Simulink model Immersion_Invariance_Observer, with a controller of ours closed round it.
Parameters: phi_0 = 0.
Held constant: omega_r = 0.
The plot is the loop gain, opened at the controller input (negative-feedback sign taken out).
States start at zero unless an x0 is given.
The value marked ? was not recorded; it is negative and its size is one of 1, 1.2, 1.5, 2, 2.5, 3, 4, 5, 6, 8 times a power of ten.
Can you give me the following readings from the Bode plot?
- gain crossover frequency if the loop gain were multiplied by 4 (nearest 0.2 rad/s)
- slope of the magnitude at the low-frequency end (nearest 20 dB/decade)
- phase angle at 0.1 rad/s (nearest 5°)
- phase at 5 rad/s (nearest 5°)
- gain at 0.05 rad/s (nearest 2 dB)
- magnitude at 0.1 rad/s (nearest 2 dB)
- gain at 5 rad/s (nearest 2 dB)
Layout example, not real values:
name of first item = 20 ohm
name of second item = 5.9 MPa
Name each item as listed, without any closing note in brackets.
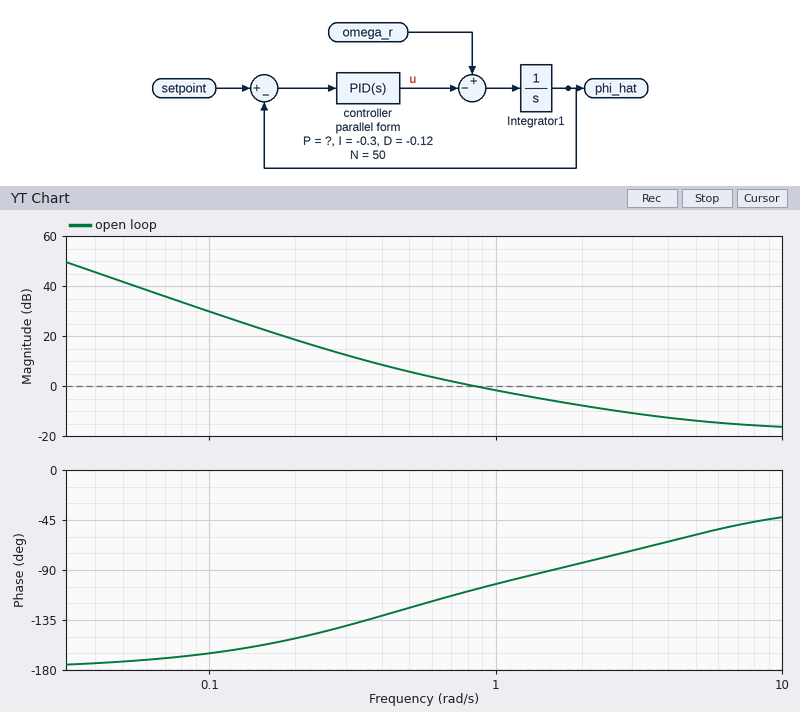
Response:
gain crossover frequency if the loop gain were multiplied by 4 = 3.6 rad/s
slope of the magnitude at the low-frequency end = -40 dB/decade
phase angle at 0.1 rad/s = -165°
phase at 5 rad/s = -60°
gain at 0.05 rad/s = 42 dB
magnitude at 0.1 rad/s = 30 dB
gain at 5 rad/s = -14 dB
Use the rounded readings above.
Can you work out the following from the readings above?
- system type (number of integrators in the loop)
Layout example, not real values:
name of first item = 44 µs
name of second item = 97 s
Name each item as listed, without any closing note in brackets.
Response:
system type = 2
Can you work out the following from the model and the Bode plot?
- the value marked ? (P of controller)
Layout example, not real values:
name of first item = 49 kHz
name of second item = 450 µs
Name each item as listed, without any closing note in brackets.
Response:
the value marked ? = -0.8
